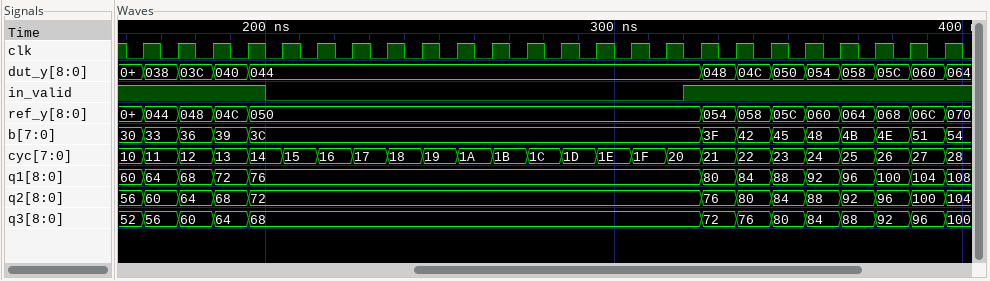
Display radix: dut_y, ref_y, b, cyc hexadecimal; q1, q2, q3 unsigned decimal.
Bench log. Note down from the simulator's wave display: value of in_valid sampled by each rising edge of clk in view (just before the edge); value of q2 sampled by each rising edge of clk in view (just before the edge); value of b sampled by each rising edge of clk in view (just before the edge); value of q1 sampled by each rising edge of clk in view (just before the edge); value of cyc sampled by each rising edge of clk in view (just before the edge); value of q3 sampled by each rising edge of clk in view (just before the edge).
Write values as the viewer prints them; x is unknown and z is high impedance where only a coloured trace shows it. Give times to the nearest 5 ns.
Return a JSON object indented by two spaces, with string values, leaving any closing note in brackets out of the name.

{
  "value of in_valid sampled by each rising edge of clk in view": "1 1 1 1 0 0 0 0 0 0 0 0 0 0 0 0 1 1 1 1 1 1 1 1",
  "value of q2 sampled by each rising edge of clk in view": "56, 60, 64, 68, 72, 72, 72, 72, 72, 72, 72, 72, 72, 72, 72, 72, 72, 76, 80, 84, 88, 92, 96, 100",
  "value of b sampled by each rising edge of clk in view": "30, 33, 36, 39, 3C, 3C, 3C, 3C, 3C, 3C, 3C, 3C, 3C, 3C, 3C, 3C, 3C, 3F, 42, 45, 48, 4B, 4E, 51",
  "value of q1 sampled by each rising edge of clk in view": "60, 64, 68, 72, 76, 76, 76, 76, 76, 76, 76, 76, 76, 76, 76, 76, 76, 80, 84, 88, 92, 96, 100, 104",
  "value of cyc sampled by each rising edge of clk in view": "10, 11, 12, 13, 14, 15, 16, 17, 18, 19, 1A, 1B, 1C, 1D, 1E, 1F, 20, 21, 22, 23, 24, 25, 26, 27",
  "value of q3 sampled by each rising edge of clk in view": "52, 56, 60, 64, 68, 68, 68, 68, 68, 68, 68, 68, 68, 68, 68, 68, 68, 72, 76, 80, 84, 88, 92, 96"
}
